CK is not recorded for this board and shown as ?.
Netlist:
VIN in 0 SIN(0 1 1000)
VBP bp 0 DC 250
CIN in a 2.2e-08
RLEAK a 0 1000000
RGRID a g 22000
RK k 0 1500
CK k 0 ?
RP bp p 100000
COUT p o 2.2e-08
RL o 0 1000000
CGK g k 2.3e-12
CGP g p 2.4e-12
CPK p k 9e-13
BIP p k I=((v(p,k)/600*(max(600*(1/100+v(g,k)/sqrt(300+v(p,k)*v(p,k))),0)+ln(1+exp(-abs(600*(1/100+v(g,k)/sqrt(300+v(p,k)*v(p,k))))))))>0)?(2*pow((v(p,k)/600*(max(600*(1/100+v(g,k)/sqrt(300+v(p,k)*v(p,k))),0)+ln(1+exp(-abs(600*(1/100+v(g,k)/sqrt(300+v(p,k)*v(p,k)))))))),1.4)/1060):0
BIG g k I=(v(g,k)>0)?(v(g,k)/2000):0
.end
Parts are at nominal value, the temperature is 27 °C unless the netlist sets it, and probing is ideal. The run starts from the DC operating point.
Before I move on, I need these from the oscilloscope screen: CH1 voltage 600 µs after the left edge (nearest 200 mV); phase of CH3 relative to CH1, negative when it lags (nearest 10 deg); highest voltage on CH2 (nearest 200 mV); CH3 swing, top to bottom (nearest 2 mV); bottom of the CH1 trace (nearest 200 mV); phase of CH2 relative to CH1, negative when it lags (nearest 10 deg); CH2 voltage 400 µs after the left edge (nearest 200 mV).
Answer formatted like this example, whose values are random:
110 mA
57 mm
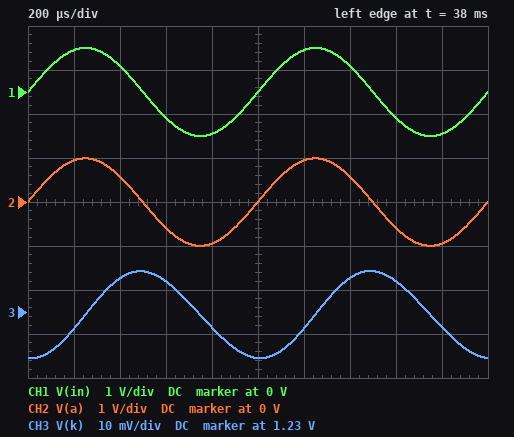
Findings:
-600 mV
-90 deg
1.0 V
20 mV
-1.0 V
0 deg
600 mV
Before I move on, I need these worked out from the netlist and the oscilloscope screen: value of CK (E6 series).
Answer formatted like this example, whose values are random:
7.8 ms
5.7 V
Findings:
10 µF
